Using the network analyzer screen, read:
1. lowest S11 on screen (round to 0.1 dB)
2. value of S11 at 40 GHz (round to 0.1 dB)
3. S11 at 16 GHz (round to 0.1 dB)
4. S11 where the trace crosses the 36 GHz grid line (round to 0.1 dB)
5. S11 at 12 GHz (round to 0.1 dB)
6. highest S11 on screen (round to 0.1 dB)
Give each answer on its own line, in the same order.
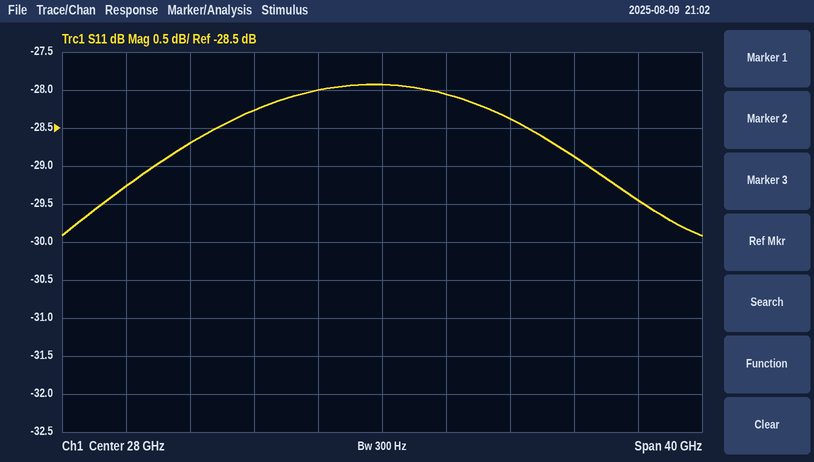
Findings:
-29.9 dB
-28.9 dB
-28.7 dB
-28.4 dB
-29.3 dB
-27.9 dB
